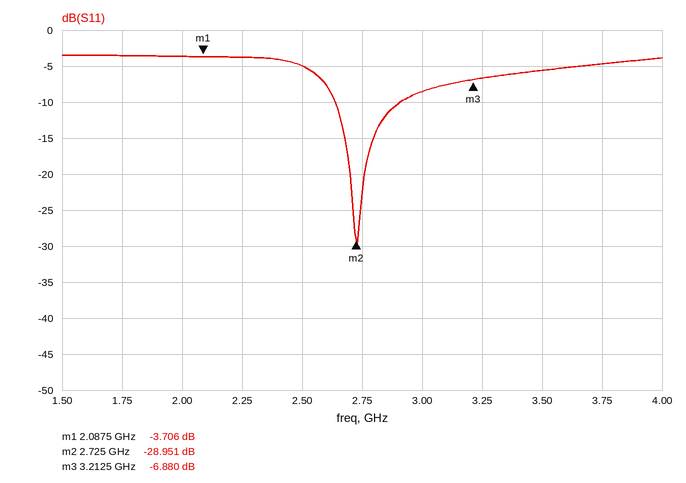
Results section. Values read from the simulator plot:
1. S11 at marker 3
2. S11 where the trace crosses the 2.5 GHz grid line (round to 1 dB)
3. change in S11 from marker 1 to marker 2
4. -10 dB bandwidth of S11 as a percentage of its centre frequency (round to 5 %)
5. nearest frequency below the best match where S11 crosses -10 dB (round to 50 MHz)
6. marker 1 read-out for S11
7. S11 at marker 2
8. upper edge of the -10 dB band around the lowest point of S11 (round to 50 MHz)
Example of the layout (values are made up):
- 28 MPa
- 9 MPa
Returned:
- -6.880 dB
- -5 dB
- -25.245 dB
- 10 %
- 2.65 GHz
- -3.706 dB
- -28.951 dB
- 2.90 GHz
